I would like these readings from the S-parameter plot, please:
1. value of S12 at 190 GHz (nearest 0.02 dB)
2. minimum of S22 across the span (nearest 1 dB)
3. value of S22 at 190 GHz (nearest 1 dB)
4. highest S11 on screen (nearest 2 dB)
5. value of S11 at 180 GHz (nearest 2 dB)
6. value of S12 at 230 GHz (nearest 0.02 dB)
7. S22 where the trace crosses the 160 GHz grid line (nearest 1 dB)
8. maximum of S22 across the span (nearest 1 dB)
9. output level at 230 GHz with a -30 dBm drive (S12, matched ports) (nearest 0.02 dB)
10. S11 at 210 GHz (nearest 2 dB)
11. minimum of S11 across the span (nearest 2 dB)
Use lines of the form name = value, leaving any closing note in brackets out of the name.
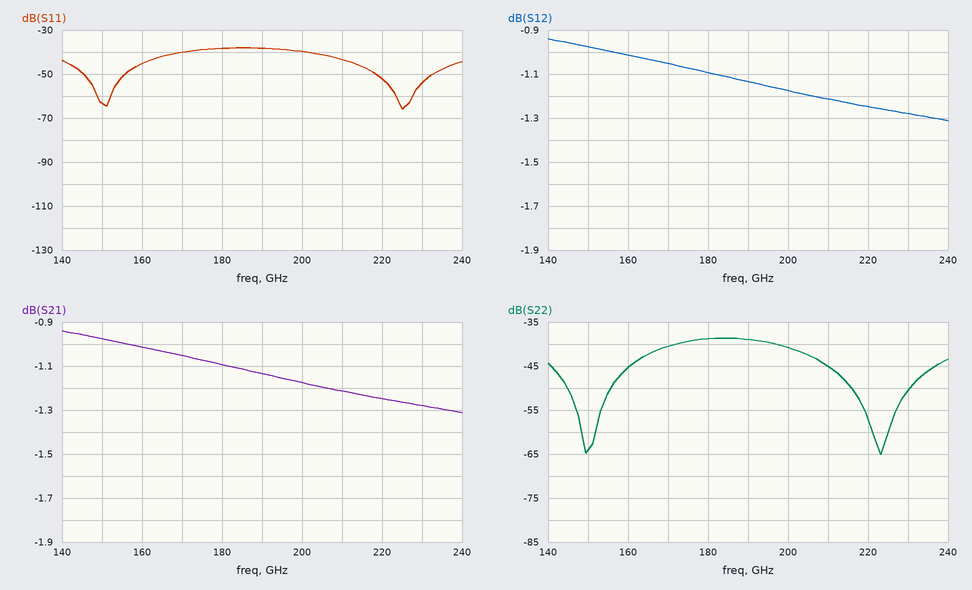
value of S12 at 190 GHz = -1.14 dB
minimum of S22 across the span = -65 dB
value of S22 at 190 GHz = -39 dB
highest S11 on screen = -38 dB
value of S11 at 180 GHz = -38 dB
value of S12 at 230 GHz = -1.28 dB
S22 where the trace crosses the 160 GHz grid line = -45 dB
maximum of S22 across the span = -39 dB
output level at 230 GHz with a -30 dBm drive (S12, matched ports) = -31.28 dBm
S11 at 210 GHz = -44 dB
minimum of S11 across the span = -66 dB
